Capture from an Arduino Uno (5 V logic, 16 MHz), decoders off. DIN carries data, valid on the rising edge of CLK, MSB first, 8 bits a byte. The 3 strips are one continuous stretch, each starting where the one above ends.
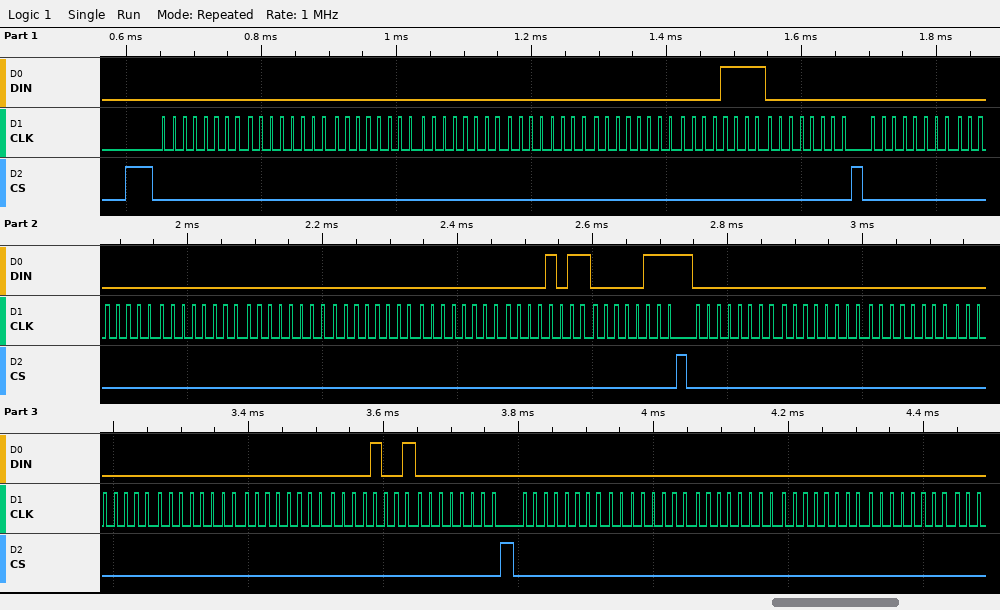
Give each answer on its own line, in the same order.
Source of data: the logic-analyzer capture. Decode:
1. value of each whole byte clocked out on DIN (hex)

0x00 0x00 0x00 0x00 0x00 0x00 0x0F 0x00 0x00 0x00 0x00 0x00 0x00 0x00 0x0B 0x07 0x00 0x00 0x00 0x00 0x00 0x00 0x09 0x00 0x00 0x00 0x00 0x00 0x00
